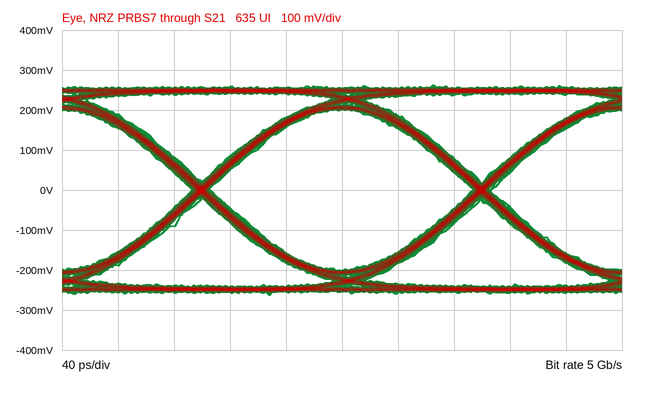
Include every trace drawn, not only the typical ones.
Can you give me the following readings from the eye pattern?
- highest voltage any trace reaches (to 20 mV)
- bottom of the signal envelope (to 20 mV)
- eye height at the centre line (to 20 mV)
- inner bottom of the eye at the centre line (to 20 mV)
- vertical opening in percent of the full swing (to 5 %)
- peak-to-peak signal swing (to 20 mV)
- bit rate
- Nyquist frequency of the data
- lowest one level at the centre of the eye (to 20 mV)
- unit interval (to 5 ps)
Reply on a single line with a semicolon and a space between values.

260 mV; -260 mV; 400 mV; -200 mV; 75 %; 520 mV; 5 Gb/s; 2.5 GHz; 200 mV; 200 ps
